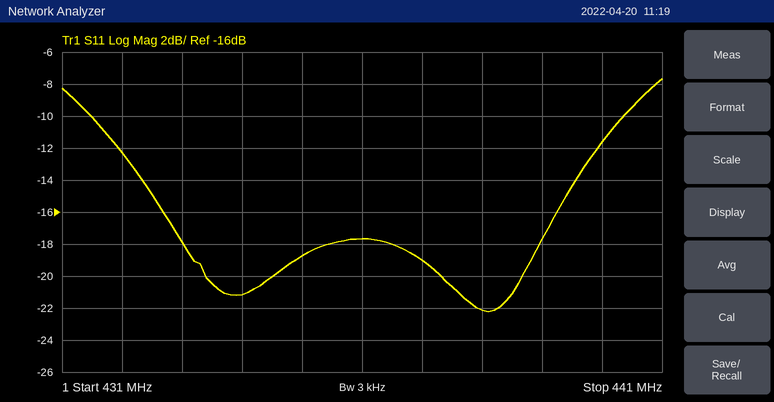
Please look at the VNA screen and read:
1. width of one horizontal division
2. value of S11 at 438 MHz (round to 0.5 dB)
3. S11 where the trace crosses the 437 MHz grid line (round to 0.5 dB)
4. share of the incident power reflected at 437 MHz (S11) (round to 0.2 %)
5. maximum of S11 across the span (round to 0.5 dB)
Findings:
1 MHz
-22.0 dB
-19.0 dB
1.2 %
-7.5 dB
